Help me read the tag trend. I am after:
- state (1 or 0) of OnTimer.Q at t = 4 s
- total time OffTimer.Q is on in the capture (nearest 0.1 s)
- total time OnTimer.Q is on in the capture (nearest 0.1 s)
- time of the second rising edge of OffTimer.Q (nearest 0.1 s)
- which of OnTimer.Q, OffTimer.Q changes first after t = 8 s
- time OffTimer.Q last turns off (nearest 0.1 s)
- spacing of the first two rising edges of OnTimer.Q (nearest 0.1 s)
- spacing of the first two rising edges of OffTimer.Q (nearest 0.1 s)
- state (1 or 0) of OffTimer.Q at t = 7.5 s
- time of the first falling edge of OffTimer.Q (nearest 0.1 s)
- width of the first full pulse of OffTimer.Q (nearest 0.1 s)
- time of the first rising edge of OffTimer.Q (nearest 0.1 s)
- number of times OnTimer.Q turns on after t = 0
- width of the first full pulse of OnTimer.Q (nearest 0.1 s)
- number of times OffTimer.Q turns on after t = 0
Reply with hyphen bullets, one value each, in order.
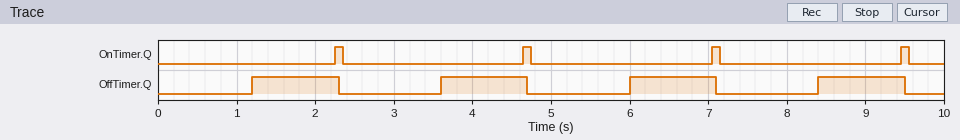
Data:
- 0
- 4.4 s
- 0.4 s
- 3.6 s
- OffTimer.Q
- 9.5 s
- 2.4 s
- 2.4 s
- 0
- 2.3 s
- 1.1 s
- 1.2 s
- 4
- 0.1 s
- 4
